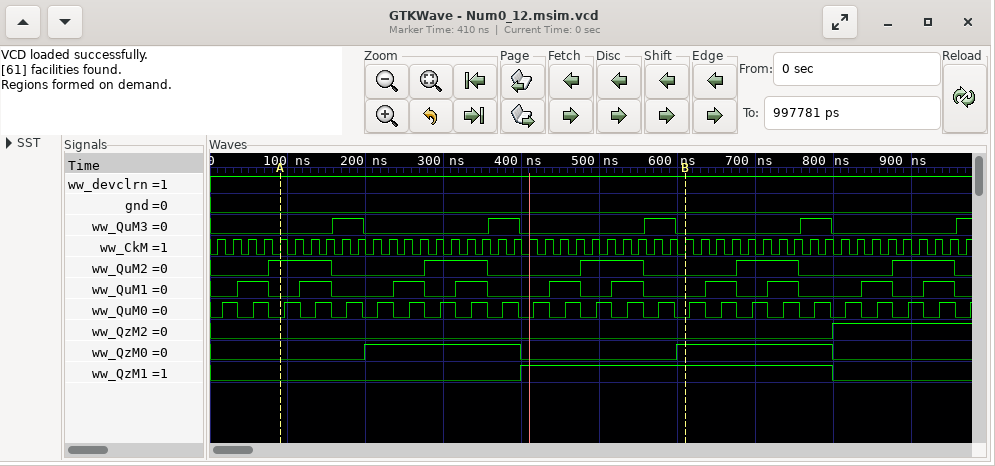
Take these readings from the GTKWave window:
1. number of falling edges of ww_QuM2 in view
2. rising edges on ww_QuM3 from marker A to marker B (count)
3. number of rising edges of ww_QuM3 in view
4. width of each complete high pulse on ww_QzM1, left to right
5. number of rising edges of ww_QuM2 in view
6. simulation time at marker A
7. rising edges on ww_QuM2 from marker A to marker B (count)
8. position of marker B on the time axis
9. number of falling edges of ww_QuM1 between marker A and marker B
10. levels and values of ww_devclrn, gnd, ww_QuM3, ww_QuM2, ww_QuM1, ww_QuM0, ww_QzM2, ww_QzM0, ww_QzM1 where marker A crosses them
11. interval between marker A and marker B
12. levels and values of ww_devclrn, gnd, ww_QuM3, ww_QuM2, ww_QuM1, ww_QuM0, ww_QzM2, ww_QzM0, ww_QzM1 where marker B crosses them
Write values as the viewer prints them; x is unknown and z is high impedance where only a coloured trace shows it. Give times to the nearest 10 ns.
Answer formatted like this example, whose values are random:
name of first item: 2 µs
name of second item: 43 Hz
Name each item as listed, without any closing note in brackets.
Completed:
number of falling edges of ww_QuM2 in view: 5
rising edges on ww_QuM3 from marker A to marker B: 3
number of rising edges of ww_QuM3 in view: 5
width of each complete high pulse on ww_QzM1, left to right: 400 ns
number of rising edges of ww_QuM2 in view: 5
simulation time at marker A: 90 ns
rising edges on ww_QuM2 from marker A to marker B: 2
position of marker B on the time axis: 610 ns
number of falling edges of ww_QuM1 between marker A and marker B: 5
levels and values of ww_devclrn, gnd, ww_QuM3, ww_QuM2, ww_QuM1, ww_QuM0, ww_QzM2, ww_QzM0, ww_QzM1 where marker A crosses them: ww_devclrn=1, gnd=0, ww_QuM3=0, ww_QuM2=1, ww_QuM1=0, ww_QuM0=0, ww_QzM2=0, ww_QzM0=0, ww_QzM1=0
interval between marker A and marker B: 520 ns
levels and values of ww_devclrn, gnd, ww_QuM3, ww_QuM2, ww_QuM1, ww_QuM0, ww_QzM2, ww_QzM0, ww_QzM1 where marker B crosses them: ww_devclrn=1, gnd=0, ww_QuM3=0, ww_QuM2=0, ww_QuM1=0, ww_QuM0=0, ww_QzM2=0, ww_QzM0=1, ww_QzM1=1
